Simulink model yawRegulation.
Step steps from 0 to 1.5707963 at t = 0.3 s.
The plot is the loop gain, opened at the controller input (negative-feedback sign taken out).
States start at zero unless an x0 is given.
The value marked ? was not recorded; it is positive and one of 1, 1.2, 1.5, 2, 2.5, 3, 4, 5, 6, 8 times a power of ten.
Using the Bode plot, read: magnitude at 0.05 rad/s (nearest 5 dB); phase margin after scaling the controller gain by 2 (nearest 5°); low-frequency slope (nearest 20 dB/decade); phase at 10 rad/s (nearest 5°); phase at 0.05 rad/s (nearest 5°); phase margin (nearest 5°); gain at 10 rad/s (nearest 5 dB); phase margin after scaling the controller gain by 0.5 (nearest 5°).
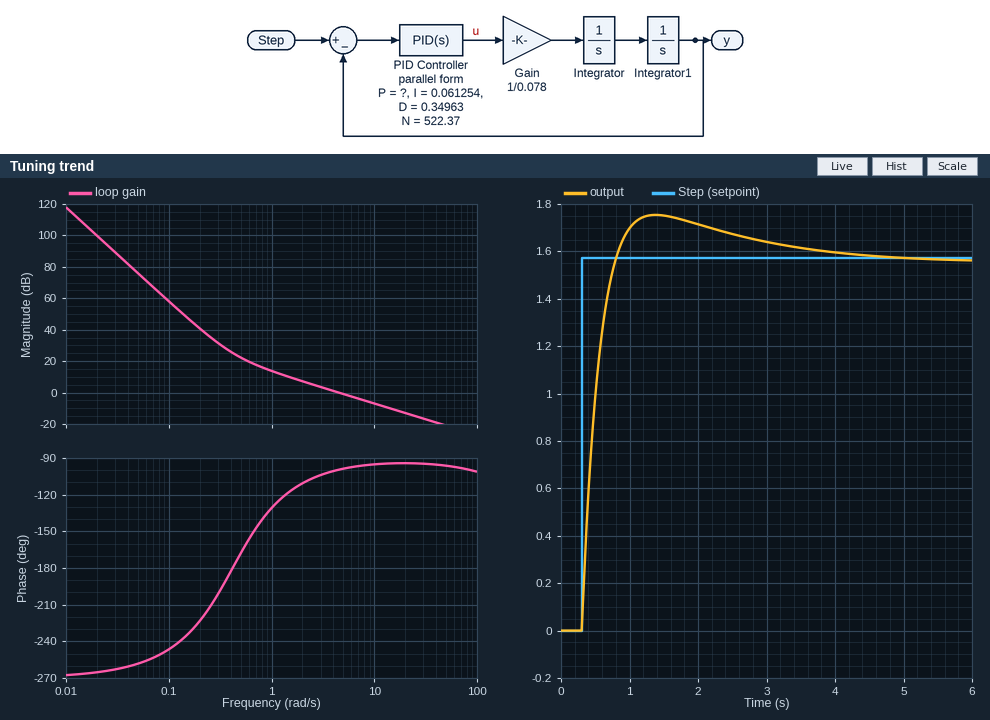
75 dB
85°
-60 dB/decade
-95°
-260°
80°
-5 dB
70°
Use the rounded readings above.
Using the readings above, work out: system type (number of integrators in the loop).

3
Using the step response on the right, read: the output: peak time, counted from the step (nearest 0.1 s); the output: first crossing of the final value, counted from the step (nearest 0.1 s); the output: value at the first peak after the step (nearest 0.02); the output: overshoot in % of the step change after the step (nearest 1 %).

1.1 s
0.5 s
1.76
12 %
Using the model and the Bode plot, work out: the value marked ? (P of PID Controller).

0.25
